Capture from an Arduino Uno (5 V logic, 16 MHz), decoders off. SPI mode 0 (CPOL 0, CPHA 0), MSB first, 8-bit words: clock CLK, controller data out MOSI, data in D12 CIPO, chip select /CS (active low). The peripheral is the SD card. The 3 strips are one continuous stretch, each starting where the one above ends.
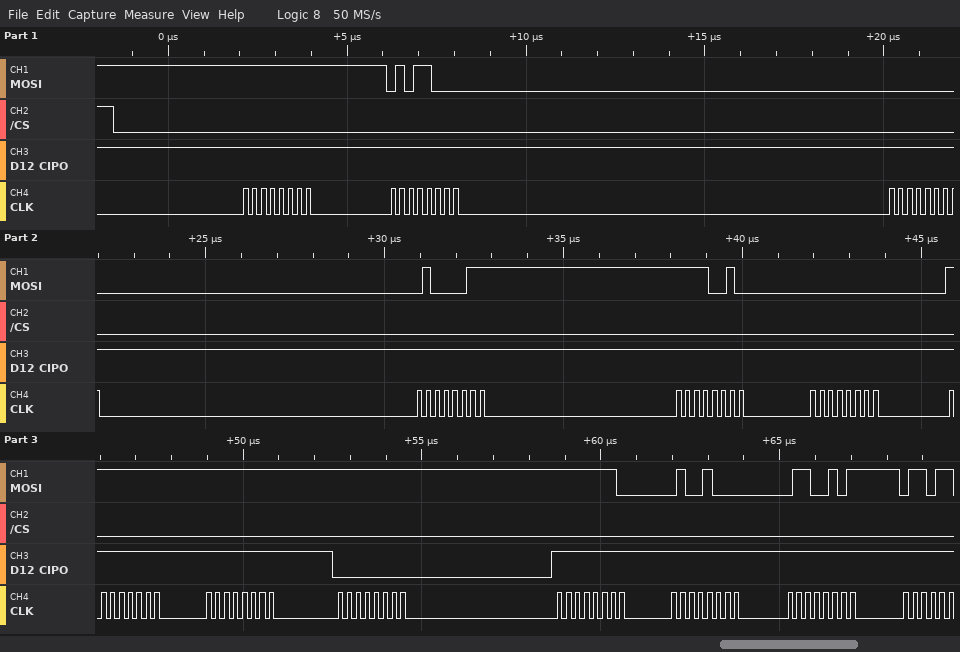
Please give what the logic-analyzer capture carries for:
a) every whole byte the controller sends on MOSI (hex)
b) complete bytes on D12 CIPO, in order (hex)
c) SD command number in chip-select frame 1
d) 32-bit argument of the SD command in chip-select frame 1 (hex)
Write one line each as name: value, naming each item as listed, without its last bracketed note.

every whole byte the controller sends on MOSI: FF 58 00 43 F2 00 FF FF FF FE 48 65
complete bytes on D12 CIPO, in order: FF FF FF FF FF FF FF FF 00 FF FF FF
SD command number in chip-select frame 1: CMD24
32-bit argument of the SD command in chip-select frame 1: 0x0043F200
